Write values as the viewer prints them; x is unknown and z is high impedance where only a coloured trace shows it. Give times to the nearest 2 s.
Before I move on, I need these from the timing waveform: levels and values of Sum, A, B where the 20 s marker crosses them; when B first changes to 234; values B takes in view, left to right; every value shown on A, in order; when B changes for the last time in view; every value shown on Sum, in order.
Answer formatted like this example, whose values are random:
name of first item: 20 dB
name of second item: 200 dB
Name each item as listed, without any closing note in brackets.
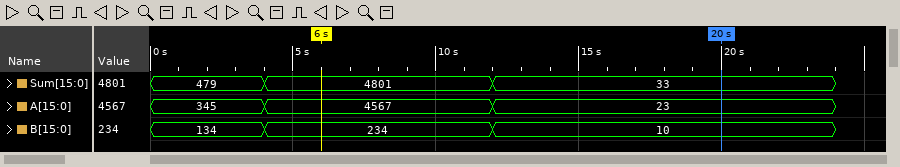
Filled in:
levels and values of Sum, A, B where the 20 s marker crosses them: Sum=33, A=23, B=10
when B first changes to 234: 4 s
values B takes in view, left to right: 134, 234, 10
every value shown on A, in order: 345, 4567, 23
when B changes for the last time in view: 12 s
every value shown on Sum, in order: 479, 4801, 33
